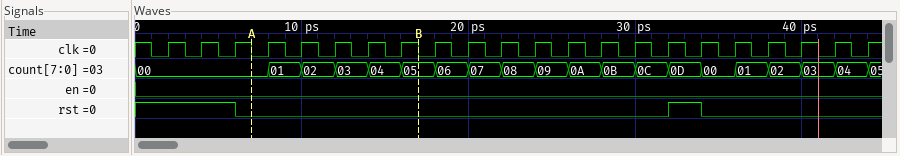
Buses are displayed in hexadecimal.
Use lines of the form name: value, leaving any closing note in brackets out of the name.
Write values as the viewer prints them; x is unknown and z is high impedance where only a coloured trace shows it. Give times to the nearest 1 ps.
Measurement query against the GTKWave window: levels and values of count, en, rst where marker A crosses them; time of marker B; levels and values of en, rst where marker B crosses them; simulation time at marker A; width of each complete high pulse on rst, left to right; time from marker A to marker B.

levels and values of count, en, rst where marker A crosses them: count=00, en=0, rst=0
time of marker B: 17 ps
levels and values of en, rst where marker B crosses them: en=0, rst=0
simulation time at marker A: 7 ps
width of each complete high pulse on rst, left to right: 2 ps
time from marker A to marker B: 10 ps
